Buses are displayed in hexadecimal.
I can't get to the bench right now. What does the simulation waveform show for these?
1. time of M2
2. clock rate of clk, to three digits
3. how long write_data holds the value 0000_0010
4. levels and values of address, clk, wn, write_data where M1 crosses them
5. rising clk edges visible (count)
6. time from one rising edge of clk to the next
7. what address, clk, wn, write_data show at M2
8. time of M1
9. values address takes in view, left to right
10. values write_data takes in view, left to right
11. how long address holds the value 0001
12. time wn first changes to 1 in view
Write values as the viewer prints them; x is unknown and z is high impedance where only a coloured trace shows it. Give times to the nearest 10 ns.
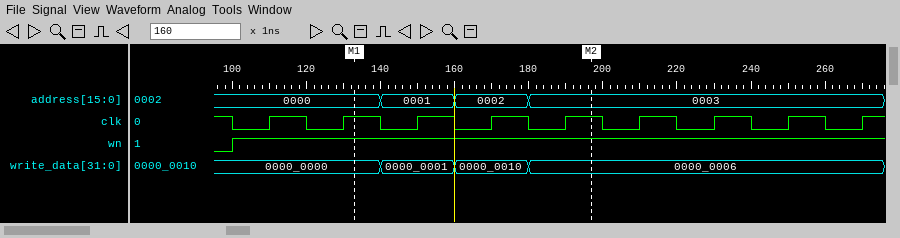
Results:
200 ns
50.0 MHz
20 ns
address=0000, clk=1, wn=1, write_data=0000_0000
9
20 ns
address=0003, clk=1, wn=1, write_data=0000_0006
130 ns
0000, 0001, 0002, 0003
0000_0000, 0000_0001, 0000_0010, 0000_0006
20 ns
100 ns
